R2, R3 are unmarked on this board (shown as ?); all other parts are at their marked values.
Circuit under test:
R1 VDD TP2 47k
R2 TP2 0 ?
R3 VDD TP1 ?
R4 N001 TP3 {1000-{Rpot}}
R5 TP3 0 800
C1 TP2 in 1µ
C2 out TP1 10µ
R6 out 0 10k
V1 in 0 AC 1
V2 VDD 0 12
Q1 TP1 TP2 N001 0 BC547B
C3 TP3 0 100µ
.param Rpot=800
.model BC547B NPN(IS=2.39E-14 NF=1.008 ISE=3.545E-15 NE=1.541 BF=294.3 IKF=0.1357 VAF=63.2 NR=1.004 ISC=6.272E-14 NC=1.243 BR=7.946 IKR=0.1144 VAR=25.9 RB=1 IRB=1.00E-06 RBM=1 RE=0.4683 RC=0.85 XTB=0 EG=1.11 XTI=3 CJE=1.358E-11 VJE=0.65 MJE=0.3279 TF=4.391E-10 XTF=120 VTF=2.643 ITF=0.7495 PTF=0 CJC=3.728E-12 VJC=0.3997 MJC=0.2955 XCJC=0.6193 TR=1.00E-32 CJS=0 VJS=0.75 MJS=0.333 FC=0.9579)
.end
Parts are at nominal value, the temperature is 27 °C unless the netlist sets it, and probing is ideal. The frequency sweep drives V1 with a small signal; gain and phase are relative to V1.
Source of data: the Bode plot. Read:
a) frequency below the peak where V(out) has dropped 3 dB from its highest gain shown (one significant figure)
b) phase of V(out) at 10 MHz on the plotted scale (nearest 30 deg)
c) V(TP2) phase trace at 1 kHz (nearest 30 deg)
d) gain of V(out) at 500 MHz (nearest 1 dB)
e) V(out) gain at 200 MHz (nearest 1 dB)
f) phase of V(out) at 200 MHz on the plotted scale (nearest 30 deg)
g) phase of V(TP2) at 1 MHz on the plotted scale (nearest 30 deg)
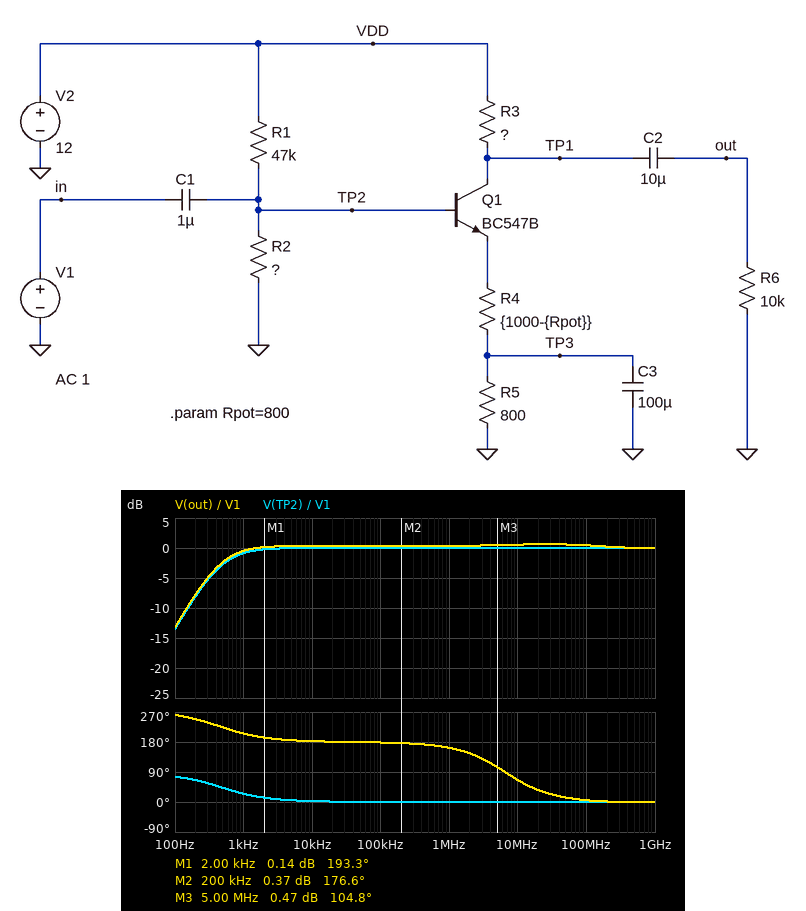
500 Hz
60 deg
30 deg
0 dB
0 dB
0 deg
0 deg
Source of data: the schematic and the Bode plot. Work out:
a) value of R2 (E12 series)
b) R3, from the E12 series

10 kΩ
10 kΩ
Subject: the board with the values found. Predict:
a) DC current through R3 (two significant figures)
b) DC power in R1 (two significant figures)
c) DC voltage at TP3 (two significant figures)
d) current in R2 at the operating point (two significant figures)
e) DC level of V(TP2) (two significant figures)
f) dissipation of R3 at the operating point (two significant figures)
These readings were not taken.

1.1 mA
2.2 mW
900 mV
180 µA
1.8 V
12 mW
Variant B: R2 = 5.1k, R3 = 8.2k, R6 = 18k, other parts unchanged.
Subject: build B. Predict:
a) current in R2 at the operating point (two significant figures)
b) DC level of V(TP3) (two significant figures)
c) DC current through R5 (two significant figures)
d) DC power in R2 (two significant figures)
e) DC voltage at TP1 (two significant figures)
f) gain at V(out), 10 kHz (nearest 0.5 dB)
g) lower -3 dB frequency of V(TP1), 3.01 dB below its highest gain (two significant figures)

230 µA
440 mV
550 µA
270 µW
7.5 V
27.0 dB
39 Hz
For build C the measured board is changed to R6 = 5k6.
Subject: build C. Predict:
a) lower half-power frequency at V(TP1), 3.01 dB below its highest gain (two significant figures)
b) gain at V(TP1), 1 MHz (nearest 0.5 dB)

520 Hz
0 dB
